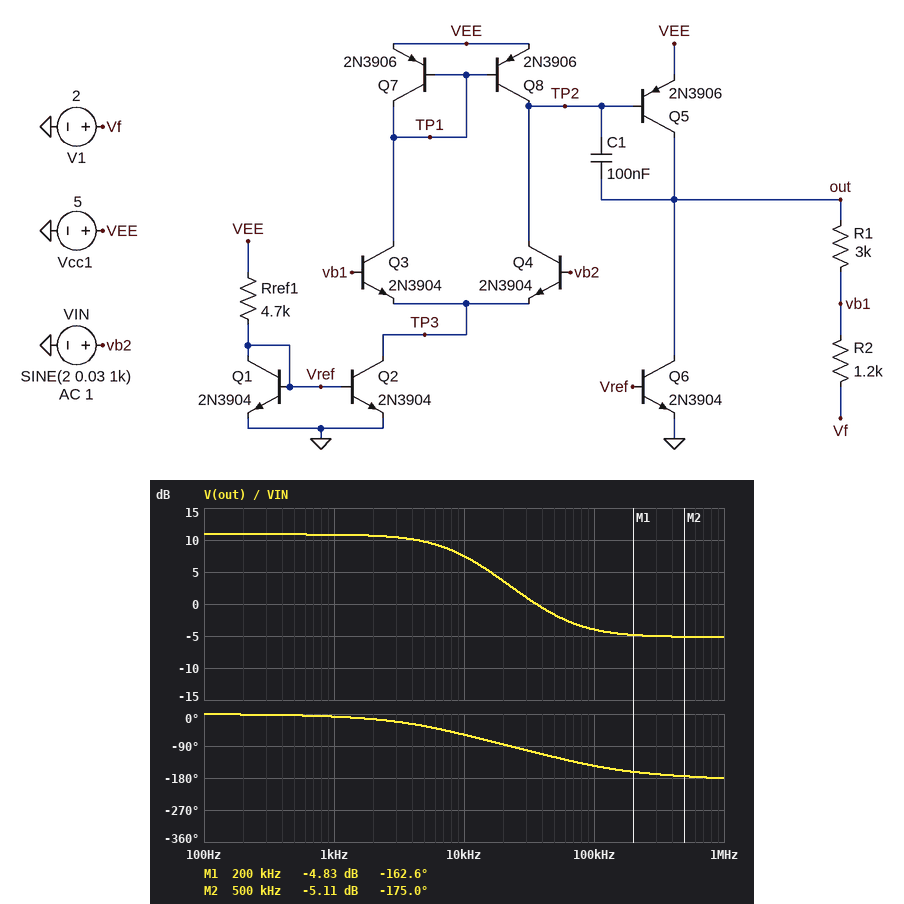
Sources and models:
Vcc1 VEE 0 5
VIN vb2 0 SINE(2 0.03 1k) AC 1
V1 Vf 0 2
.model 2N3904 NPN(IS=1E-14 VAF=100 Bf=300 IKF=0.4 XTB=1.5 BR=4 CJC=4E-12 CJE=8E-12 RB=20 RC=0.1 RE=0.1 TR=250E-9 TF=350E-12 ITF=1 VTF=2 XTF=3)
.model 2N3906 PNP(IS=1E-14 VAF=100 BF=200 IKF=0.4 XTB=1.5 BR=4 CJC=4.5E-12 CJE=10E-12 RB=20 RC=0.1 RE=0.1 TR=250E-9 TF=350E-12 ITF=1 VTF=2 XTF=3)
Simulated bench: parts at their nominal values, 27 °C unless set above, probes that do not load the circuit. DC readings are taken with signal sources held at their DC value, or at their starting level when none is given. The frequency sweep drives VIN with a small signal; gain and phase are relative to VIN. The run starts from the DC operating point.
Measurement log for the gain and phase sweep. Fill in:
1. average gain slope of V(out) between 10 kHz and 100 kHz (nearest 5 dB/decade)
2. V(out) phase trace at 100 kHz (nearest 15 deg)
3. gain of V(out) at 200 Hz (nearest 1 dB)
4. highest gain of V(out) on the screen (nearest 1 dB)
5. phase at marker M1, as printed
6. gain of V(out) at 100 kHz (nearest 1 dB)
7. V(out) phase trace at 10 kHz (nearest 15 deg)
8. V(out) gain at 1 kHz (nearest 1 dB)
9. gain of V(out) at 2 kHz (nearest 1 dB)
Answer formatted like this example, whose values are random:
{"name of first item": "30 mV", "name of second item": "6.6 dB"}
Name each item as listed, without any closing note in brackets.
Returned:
{"average gain slope of V(out) between 10 kHz and 100 kHz": "-10 dB/decade", "V(out) phase trace at 100 kHz": "-150 deg", "gain of V(out) at 200 Hz": "11 dB", "highest gain of V(out) on the screen": "11 dB", "phase at marker M1, as printed": "-162.6 deg", "gain of V(out) at 100 kHz": "-4 dB", "V(out) phase trace at 10 kHz": "-60 deg", "V(out) gain at 1 kHz": "11 dB", "gain of V(out) at 2 kHz": "11 dB"}
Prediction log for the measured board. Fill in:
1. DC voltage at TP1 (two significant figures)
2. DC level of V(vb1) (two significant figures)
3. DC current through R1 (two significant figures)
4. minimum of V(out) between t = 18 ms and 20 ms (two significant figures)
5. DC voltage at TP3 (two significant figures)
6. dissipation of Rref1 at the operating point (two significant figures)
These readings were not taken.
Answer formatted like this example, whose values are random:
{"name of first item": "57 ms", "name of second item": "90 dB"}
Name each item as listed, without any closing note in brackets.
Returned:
{"DC voltage at TP1": "4.4 V", "DC level of V(vb1)": "2.0 V", "DC current through R1": "1.5 µA", "minimum of V(out) between t = 18 ms and 20 ms": "1.9 V", "DC voltage at TP3": "1.4 V", "dissipation of Rref1 at the operating point": "4.0 mW"}
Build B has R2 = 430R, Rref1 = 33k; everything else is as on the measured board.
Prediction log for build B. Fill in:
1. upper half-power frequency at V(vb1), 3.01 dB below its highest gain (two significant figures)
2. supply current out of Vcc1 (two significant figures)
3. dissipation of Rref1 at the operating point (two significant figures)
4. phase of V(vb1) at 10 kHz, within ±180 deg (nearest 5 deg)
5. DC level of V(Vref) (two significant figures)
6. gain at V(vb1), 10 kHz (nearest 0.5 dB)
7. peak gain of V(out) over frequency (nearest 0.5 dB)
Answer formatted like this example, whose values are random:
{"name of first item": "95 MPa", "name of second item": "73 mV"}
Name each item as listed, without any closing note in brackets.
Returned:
{"upper half-power frequency at V(vb1), 3.01 dB below its highest gain": "510 Hz", "supply current out of Vcc1": "400 µA", "dissipation of Rref1 at the operating point": "590 µW", "phase of V(vb1) at 10 kHz, within ±180 deg": "-135 deg", "DC level of V(Vref)": "600 mV", "gain at V(vb1), 10 kHz": "-22.0 dB", "peak gain of V(out) over frequency": "18.0 dB"}
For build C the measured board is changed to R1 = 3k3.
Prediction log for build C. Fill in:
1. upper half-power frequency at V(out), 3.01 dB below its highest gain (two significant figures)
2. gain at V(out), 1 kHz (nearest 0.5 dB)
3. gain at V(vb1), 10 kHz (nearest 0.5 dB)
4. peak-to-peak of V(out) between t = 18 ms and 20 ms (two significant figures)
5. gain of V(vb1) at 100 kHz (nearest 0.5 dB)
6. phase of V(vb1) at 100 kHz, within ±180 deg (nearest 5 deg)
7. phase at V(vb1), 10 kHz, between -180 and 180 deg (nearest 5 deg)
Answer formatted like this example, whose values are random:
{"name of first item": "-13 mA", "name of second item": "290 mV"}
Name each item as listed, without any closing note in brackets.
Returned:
{"upper half-power frequency at V(out), 3.01 dB below its highest gain": "8.4 kHz", "gain at V(out), 1 kHz": "11.5 dB", "gain at V(vb1), 10 kHz": "-4.0 dB", "peak-to-peak of V(out) between t = 18 ms and 20 ms": "220 mV", "gain of V(vb1) at 100 kHz": "-17.0 dB", "phase of V(vb1) at 100 kHz, within ±180 deg": "-145 deg", "phase at V(vb1), 10 kHz, between -180 and 180 deg": "-60 deg"}
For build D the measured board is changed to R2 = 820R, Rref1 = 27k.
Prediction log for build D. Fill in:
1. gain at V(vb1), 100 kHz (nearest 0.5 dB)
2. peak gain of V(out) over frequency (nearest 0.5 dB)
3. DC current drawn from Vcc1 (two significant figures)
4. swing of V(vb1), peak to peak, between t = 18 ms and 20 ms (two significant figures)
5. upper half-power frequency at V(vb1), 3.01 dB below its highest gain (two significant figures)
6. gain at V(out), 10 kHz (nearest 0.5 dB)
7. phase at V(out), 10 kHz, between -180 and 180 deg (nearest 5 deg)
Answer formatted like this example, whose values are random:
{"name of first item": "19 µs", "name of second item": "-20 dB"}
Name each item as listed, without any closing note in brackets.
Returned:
{"gain at V(vb1), 100 kHz": "-19.5 dB", "peak gain of V(out) over frequency": "13.5 dB", "DC current drawn from Vcc1": "490 µA", "swing of V(vb1), peak to peak, between t = 18 ms and 20 ms": "44 mV", "upper half-power frequency at V(vb1), 3.01 dB below its highest gain": "1.1 kHz", "gain at V(out), 10 kHz": "-2.5 dB", "phase at V(out), 10 kHz, between -180 and 180 deg": "-130 deg"}
